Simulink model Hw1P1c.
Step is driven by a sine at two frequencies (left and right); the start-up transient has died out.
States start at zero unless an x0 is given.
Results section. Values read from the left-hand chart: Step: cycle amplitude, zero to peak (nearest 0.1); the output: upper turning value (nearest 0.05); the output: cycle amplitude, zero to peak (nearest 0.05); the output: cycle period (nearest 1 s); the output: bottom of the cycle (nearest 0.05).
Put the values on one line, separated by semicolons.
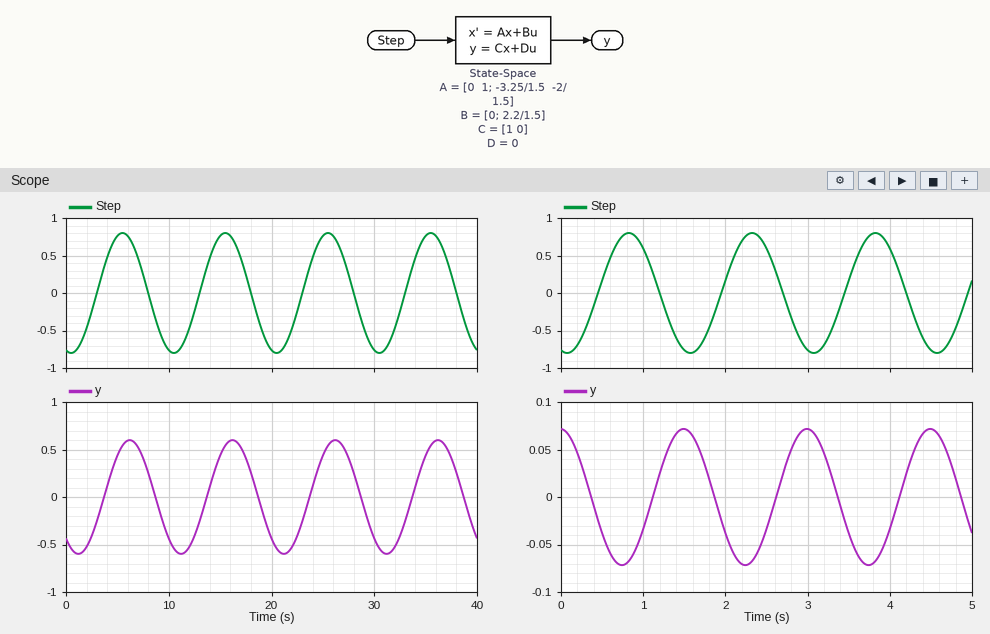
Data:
0.8; 0.60; 0.60; 10 s; -0.60
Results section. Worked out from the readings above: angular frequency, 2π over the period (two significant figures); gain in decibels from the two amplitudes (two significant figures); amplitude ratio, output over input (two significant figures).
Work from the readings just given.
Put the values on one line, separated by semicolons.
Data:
0.63 rad/s; -2.5 dB; 0.75
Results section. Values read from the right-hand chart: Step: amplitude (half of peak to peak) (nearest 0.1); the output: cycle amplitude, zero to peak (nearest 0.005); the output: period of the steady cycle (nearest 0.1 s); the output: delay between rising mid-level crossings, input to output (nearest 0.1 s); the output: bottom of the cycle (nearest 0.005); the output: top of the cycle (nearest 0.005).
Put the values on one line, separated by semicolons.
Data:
0.8; 0.070; 1.5 s; 0.7 s; -0.070; 0.070
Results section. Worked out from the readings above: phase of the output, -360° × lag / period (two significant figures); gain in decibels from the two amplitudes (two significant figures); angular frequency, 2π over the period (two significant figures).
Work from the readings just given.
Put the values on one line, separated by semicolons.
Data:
-170°; -21 dB; 4.2 rad/s
